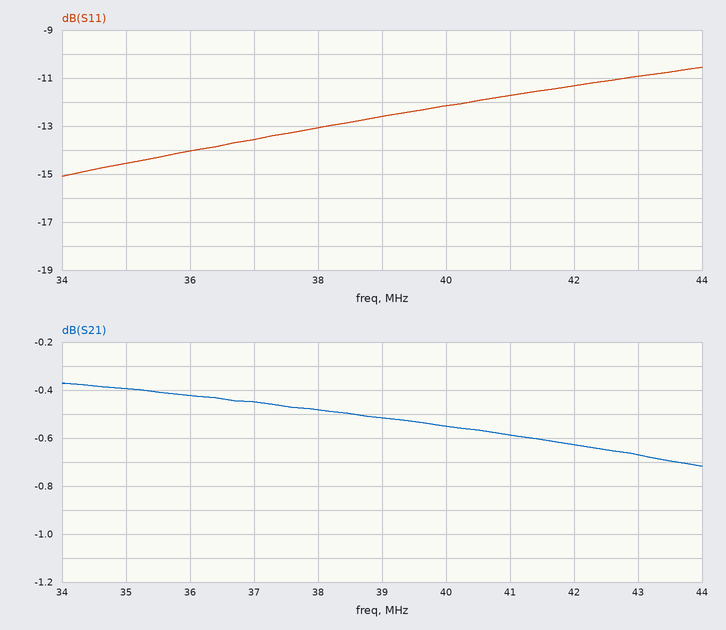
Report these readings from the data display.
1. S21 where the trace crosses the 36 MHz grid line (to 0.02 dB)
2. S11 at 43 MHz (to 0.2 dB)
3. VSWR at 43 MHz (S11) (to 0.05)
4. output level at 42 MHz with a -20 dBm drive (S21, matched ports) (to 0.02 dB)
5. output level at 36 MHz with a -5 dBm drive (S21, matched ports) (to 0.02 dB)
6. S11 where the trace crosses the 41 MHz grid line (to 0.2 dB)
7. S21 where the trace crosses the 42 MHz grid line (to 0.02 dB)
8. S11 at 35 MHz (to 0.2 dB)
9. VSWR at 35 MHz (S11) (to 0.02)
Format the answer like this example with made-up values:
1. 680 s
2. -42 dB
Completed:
1. -0.42 dB
2. -11.0 dB
3. 1.80
4. -20.62 dBm
5. -5.42 dBm
6. -11.8 dB
7. -0.62 dB
8. -14.6 dB
9. 1.46
